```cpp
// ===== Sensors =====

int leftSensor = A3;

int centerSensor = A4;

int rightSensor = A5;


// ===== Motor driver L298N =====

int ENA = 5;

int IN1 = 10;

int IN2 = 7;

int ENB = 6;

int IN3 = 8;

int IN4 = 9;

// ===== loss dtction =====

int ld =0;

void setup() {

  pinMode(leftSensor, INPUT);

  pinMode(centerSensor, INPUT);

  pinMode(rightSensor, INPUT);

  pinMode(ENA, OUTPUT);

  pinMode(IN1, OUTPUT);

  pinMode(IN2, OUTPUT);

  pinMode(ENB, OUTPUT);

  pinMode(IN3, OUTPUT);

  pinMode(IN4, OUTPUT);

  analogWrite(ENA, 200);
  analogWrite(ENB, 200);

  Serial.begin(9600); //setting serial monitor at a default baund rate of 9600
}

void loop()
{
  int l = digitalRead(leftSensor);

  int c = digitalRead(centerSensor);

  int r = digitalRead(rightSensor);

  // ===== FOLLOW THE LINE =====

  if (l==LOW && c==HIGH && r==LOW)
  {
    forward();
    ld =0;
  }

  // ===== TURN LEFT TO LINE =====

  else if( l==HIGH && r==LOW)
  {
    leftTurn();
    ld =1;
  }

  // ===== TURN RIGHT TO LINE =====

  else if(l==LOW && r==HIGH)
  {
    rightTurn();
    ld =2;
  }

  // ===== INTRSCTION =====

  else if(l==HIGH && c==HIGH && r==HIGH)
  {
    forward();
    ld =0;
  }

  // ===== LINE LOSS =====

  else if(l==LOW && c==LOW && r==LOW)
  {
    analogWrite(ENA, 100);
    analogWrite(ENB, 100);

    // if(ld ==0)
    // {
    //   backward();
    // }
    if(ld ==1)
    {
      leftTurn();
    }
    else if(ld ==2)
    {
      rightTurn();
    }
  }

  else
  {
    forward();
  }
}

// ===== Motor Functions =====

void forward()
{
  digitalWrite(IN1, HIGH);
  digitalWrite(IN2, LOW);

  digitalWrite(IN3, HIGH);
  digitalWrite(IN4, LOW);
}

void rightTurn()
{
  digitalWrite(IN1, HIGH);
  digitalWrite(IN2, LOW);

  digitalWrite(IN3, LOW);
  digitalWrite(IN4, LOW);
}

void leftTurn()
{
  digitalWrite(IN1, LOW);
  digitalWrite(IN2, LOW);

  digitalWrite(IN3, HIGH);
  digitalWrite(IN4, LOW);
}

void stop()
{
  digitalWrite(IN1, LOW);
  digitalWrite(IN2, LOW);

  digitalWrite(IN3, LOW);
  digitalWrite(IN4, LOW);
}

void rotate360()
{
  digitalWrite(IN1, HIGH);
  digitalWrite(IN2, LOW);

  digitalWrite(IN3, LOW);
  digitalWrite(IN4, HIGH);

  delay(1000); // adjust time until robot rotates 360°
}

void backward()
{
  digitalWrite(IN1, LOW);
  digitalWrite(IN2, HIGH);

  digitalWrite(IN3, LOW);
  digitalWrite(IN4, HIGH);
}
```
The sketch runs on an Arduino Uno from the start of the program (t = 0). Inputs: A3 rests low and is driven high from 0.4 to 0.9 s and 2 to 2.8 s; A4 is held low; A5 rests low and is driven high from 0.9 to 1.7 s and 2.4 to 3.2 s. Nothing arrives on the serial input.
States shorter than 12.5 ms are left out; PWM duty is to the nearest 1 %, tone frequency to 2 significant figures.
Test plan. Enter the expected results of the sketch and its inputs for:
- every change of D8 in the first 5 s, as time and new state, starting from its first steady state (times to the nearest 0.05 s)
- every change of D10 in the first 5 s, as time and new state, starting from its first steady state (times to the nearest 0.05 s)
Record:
0 s low; 0.4 s high; 0.9 s low; 2 s high; 2.8 s low
0 s low; 0.9 s high; 2 s low; 2.4 s high
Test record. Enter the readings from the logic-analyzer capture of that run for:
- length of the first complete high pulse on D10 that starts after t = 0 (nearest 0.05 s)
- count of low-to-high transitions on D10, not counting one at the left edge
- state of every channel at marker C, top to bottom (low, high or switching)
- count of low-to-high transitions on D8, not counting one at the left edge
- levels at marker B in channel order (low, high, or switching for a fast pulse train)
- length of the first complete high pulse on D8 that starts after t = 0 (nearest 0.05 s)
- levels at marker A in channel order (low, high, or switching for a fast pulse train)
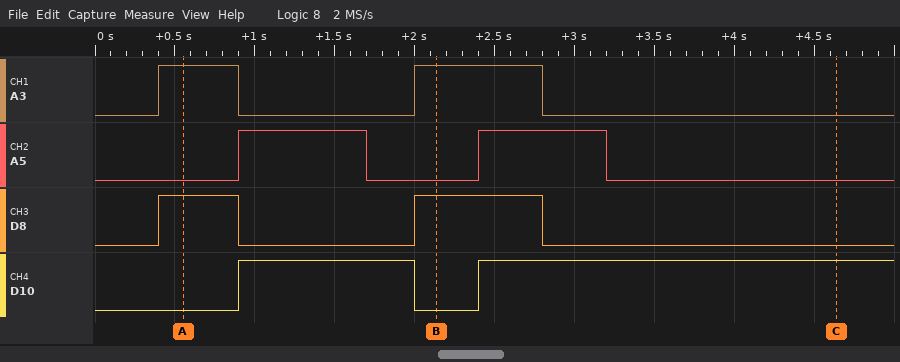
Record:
1.10 s
2
A3 low, A5 low, D8 low, D10 high
2
A3 high, A5 low, D8 high, D10 low
0.50 s
A3 high, A5 low, D8 high, D10 low
